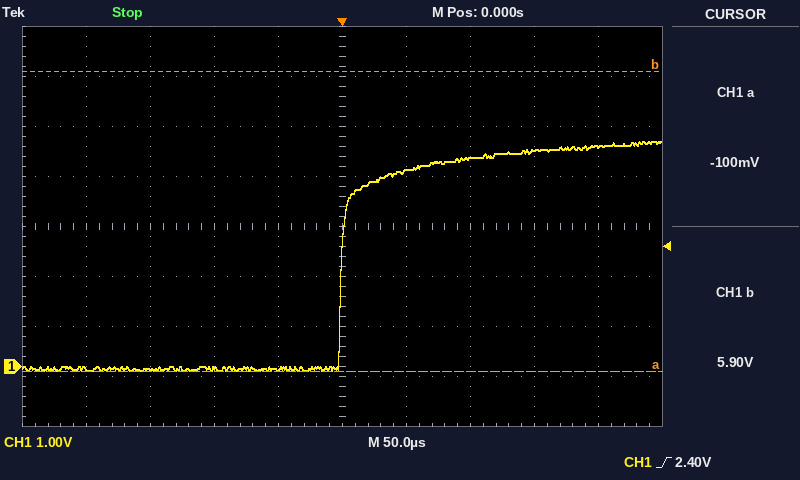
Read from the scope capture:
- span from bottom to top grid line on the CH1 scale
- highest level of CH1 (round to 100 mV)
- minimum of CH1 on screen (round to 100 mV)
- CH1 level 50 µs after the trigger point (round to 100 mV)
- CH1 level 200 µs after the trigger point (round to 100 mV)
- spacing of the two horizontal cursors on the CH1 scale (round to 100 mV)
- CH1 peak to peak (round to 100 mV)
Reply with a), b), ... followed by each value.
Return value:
a) 8 V
b) 4.5 V
c) -100 mV
d) 3.9 V
e) 4.4 V
f) 6.0 V
g) 4.6 V
